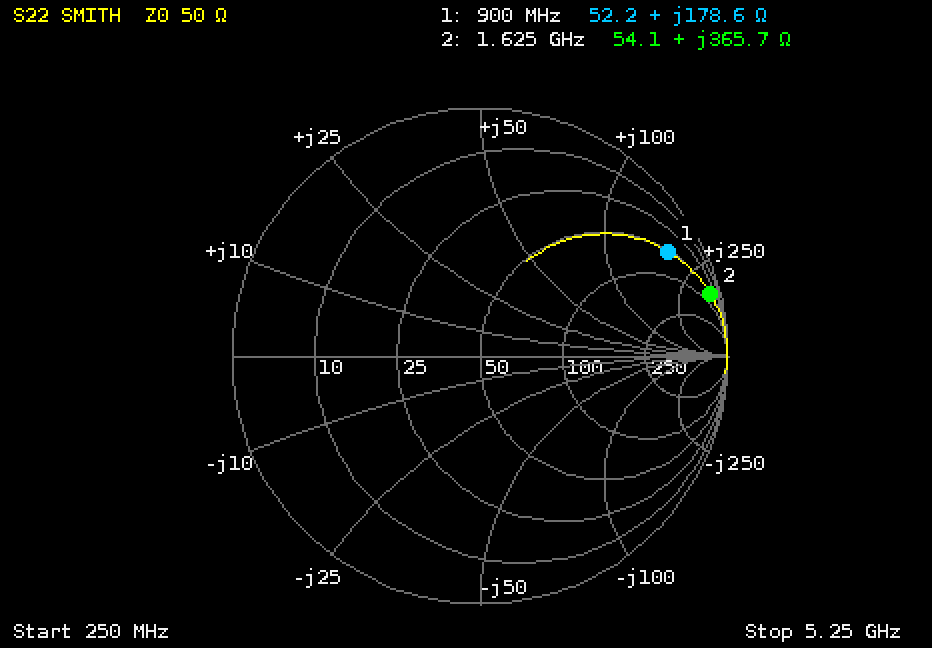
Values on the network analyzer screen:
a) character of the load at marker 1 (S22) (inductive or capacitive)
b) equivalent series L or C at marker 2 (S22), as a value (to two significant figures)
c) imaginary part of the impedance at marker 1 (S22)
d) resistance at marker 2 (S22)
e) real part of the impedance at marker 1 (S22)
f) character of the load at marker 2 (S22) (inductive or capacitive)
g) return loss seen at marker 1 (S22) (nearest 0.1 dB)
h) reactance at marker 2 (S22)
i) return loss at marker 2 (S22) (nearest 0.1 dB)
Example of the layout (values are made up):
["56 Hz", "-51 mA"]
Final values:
["inductive", "36 nH", "+178.6 Ω", "54.1 Ω", "52.2 Ω", "inductive", "1.2 dB", "+365.7 Ω", "0.3 dB"]
